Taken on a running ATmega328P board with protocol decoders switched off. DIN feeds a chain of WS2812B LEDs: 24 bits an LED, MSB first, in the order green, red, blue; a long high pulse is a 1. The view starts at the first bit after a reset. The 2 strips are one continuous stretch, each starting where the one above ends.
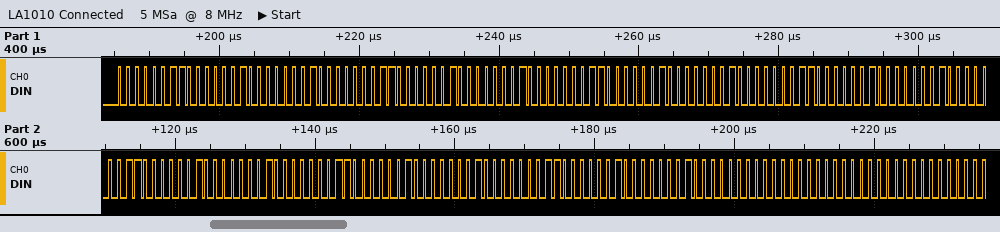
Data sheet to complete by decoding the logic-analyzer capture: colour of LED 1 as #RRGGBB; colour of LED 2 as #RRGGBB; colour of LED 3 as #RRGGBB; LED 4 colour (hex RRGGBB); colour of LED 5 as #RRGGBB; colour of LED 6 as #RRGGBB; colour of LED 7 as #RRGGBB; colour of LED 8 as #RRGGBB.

#020302
#020302
#020302
#020302
#020302
#020302
#020302
#000000
